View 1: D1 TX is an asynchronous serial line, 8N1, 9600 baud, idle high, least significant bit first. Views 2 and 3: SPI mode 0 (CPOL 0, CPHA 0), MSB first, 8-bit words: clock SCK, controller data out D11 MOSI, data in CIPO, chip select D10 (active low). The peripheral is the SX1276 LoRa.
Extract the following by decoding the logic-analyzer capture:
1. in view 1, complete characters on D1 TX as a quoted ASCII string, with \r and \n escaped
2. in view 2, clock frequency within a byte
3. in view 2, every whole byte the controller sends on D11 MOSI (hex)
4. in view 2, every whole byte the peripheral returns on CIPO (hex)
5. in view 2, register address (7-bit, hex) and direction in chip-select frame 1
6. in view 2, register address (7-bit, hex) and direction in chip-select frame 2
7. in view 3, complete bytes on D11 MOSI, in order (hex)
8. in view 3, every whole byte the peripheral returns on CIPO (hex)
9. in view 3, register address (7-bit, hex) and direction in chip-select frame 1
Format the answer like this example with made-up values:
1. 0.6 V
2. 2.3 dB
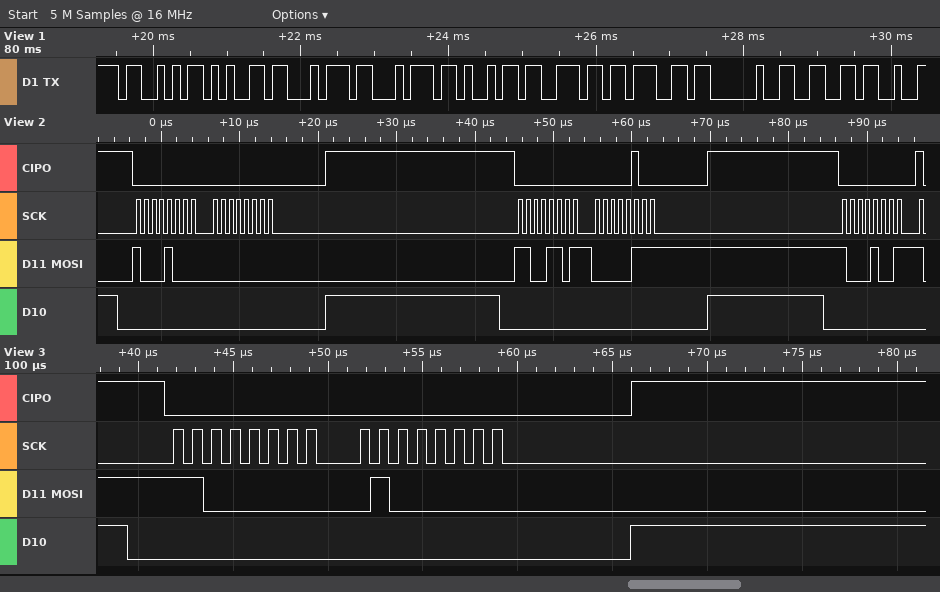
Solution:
1. "Setting f"
2. 1 MHz
3. 88 00 CD 07 89
4. 00 00 00 04 00
5. 0x08 write
6. 0x4D write
7. C0 40
8. 00 00
9. 0x40 write
